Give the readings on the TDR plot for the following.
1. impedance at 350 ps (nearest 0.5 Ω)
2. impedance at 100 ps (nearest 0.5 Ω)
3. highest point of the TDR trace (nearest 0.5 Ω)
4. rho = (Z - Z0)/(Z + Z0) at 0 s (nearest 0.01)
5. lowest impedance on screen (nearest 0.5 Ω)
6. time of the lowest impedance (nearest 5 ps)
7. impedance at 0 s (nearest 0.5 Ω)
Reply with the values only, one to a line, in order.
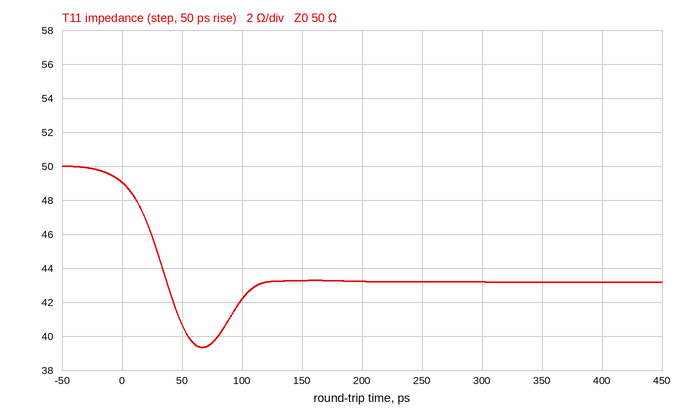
43.0 Ω
42.0 Ω
50.0 Ω
-0.01
39.5 Ω
65 ps
49.0 Ω
